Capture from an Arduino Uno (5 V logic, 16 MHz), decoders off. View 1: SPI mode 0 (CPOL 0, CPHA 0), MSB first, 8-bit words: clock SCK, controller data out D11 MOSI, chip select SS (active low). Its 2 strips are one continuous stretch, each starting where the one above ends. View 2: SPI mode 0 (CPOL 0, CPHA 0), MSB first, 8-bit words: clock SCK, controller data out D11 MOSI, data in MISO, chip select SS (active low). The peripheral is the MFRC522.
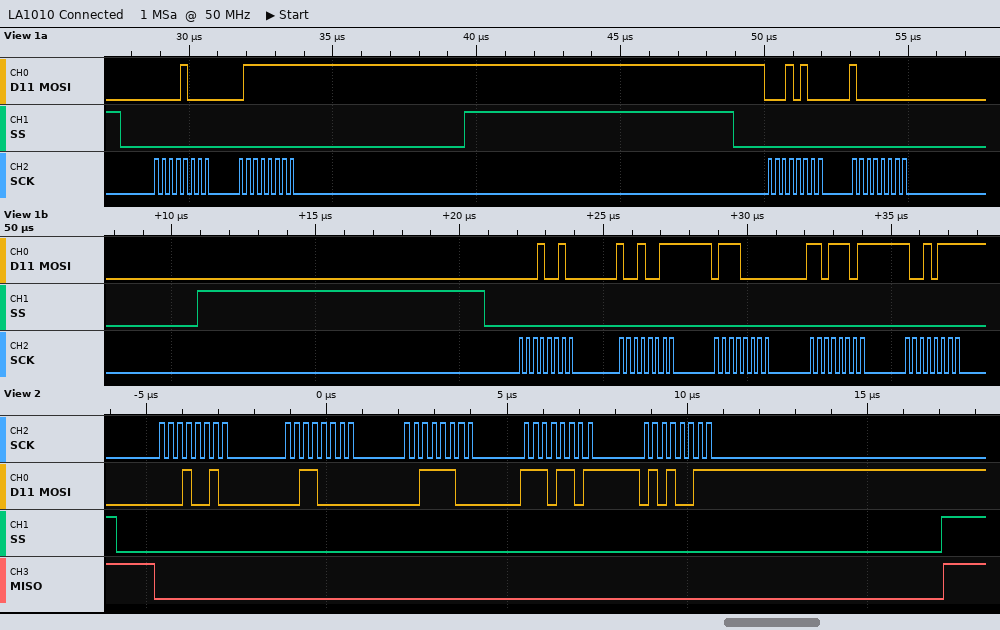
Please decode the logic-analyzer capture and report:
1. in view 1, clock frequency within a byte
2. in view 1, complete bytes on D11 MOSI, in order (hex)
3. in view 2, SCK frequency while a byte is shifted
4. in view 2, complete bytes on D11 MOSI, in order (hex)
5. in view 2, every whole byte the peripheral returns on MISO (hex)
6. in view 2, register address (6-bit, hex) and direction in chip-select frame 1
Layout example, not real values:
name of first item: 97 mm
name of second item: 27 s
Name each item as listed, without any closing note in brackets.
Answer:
in view 1, clock frequency within a byte: 4 MHz
in view 1, complete bytes on D11 MOSI, in order: 08 7F 14 80 12 93 70 DD 97
in view 2, SCK frequency while a byte is shifted: 4 MHz
in view 2, complete bytes on D11 MOSI, in order: 12 30 3C ED 53
in view 2, every whole byte the peripheral returns on MISO: 00 00 00 00 00
in view 2, register address (6-bit, hex) and direction in chip-select frame 1: 0x09 write
